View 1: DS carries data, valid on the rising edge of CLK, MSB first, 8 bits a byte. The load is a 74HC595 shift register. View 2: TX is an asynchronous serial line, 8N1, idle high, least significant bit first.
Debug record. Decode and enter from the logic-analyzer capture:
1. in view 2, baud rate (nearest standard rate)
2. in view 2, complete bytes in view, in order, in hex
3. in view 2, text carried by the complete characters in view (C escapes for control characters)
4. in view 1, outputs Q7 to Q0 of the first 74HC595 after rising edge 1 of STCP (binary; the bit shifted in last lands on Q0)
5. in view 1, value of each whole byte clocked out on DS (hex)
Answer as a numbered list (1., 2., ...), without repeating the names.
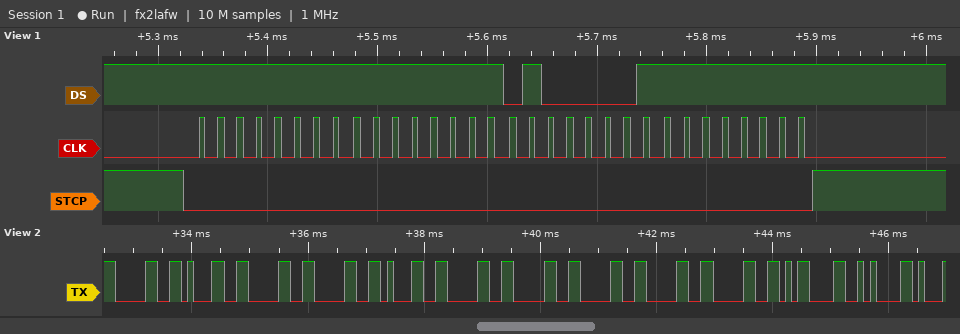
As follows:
1. 9600 baud
2. 30 31 30 30 31 30 30 30 30 30 0D 0A
3. "0100100000\r\n"
4. 11111111
5. FF FF 41 FF
